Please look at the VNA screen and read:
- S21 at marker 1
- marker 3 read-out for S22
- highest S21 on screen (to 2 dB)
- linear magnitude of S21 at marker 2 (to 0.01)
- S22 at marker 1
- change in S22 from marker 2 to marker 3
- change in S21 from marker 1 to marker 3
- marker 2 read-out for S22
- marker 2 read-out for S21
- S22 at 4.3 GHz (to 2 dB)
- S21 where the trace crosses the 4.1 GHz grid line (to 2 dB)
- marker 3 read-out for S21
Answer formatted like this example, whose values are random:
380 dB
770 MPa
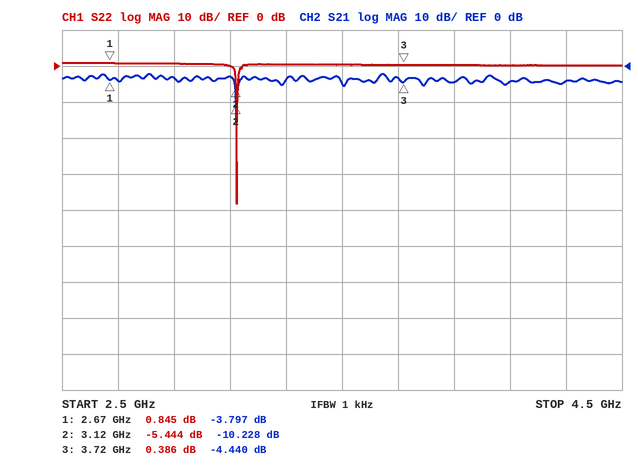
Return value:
-3.797 dB
0.386 dB
-2 dB
0.31
0.845 dB
5.830 dB
-0.643 dB
-5.444 dB
-10.228 dB
0 dB
-4 dB
-4.440 dB
